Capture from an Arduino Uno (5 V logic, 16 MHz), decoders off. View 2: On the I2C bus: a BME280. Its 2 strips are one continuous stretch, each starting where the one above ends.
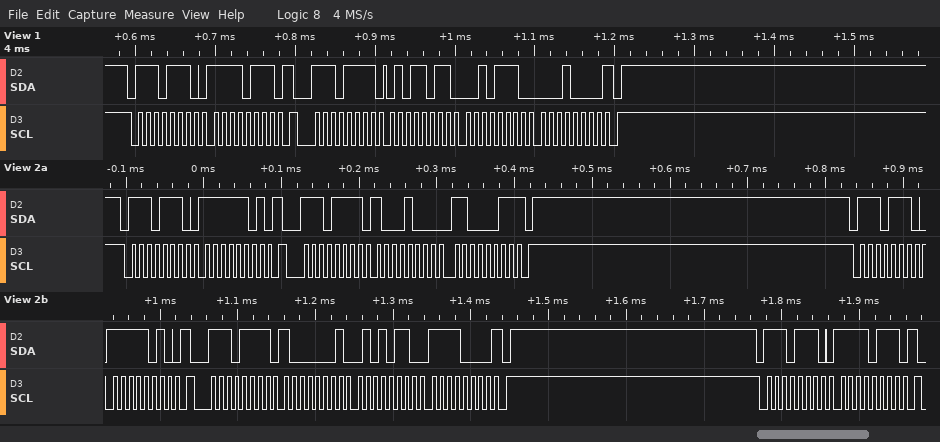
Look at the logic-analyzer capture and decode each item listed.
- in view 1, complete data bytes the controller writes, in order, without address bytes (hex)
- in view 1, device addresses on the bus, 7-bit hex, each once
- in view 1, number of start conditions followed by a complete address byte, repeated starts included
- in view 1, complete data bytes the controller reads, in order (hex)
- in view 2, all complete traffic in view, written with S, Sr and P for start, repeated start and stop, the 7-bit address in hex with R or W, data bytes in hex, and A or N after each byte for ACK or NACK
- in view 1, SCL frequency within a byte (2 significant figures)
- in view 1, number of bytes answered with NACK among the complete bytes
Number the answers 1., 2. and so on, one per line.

1. F7
2. 0x77
3. 2
4. 5B 2E 10
5. S 77W A FD A Sr 77R A 88 A C3 N P S 77W A FA A Sr 77R A 81 A 56 A F0 N P S 77W A F7 A
6. 100 kHz
7. 1
